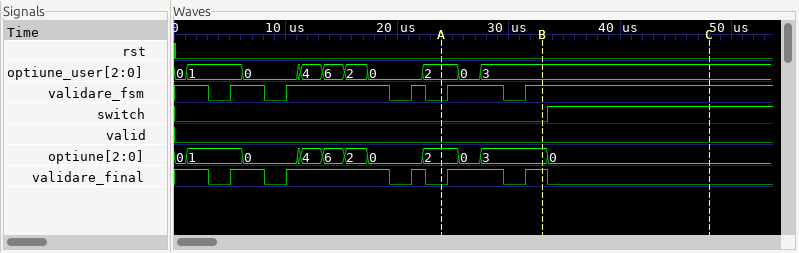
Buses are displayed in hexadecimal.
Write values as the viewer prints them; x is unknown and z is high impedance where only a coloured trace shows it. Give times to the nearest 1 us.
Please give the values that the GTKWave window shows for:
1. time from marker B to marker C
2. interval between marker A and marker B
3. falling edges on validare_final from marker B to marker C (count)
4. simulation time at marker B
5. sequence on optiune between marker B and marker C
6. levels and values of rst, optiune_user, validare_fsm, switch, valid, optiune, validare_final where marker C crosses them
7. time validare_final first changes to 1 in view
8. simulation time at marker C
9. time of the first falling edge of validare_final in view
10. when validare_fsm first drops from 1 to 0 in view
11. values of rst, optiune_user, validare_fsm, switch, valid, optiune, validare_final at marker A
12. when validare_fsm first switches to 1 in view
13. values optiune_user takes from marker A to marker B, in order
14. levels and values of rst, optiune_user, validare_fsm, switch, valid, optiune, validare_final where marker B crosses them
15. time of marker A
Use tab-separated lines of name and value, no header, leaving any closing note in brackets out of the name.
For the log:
time from marker B to marker C	15 us
interval between marker A and marker B	9 us
falling edges on validare_final from marker B to marker C	1
simulation time at marker B	33 us
sequence on optiune between marker B and marker C	3, 0
levels and values of rst, optiune_user, validare_fsm, switch, valid, optiune, validare_final where marker C crosses them	rst=0, optiune_user=3, validare_fsm=1, switch=1, valid=0, optiune=0, validare_final=0
time validare_final first changes to 1 in view	5 us
simulation time at marker C	48 us
time of the first falling edge of validare_final in view	3 us
when validare_fsm first drops from 1 to 0 in view	3 us
values of rst, optiune_user, validare_fsm, switch, valid, optiune, validare_final at marker A	rst=0, optiune_user=2, validare_fsm=0, switch=0, valid=0, optiune=2, validare_final=0
when validare_fsm first switches to 1 in view	5 us
values optiune_user takes from marker A to marker B, in order	2, 0, 3
levels and values of rst, optiune_user, validare_fsm, switch, valid, optiune, validare_final where marker B crosses them	rst=0, optiune_user=3, validare_fsm=1, switch=0, valid=0, optiune=3, validare_final=1
time of marker A	24 us
